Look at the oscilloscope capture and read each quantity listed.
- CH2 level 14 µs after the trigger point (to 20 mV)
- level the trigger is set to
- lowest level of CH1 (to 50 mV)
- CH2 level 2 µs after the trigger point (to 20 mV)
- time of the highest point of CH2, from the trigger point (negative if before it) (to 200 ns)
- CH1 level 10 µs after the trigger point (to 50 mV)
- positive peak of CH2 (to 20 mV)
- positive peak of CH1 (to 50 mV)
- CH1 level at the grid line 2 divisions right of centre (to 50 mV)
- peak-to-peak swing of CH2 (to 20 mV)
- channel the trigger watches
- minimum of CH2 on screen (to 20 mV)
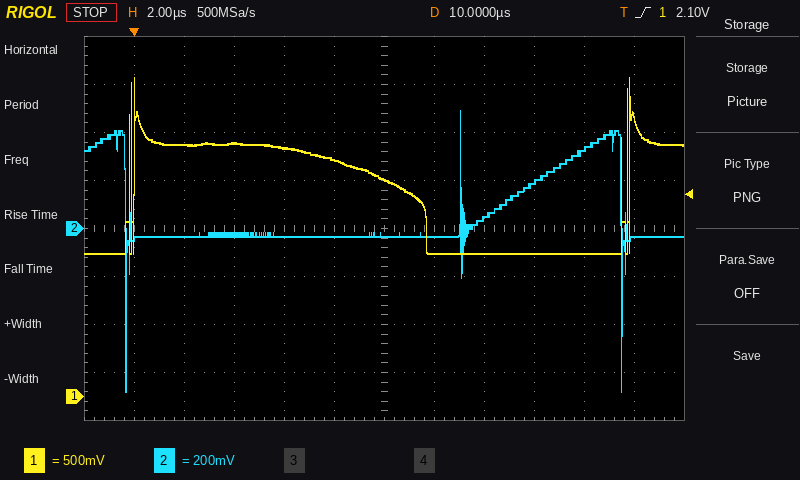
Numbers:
40 mV
2.10 V
1.50 V
-40 mV
+13.0 µs
2.25 V
500 mV
3.30 V
1.50 V
1.18 V
CH1
-680 mV
